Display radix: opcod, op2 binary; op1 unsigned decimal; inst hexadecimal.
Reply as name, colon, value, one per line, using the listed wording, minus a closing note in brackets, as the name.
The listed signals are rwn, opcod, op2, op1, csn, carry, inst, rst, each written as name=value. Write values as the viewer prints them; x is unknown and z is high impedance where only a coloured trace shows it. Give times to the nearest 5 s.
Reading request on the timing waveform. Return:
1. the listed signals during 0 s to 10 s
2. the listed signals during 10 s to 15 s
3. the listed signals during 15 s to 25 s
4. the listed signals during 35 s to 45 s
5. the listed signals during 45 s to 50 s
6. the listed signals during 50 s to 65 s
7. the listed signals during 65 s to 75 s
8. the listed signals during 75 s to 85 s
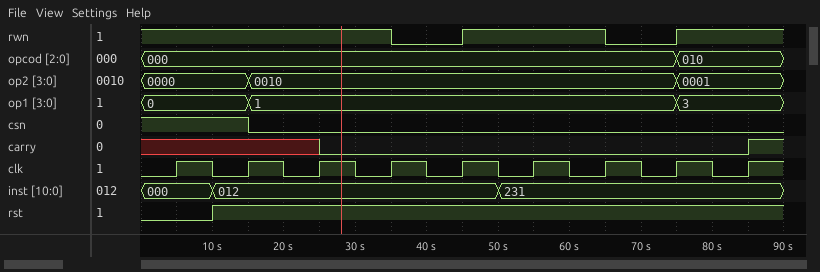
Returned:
the listed signals during 0 s to 10 s: rwn=1, opcod=000, op2=0000, op1=0, csn=1, carry=x, inst=000, rst=0
the listed signals during 10 s to 15 s: rwn=1, opcod=000, op2=0000, op1=0, csn=1, carry=x, inst=012, rst=1
the listed signals during 15 s to 25 s: rwn=1, opcod=000, op2=0010, op1=1, csn=0, carry=x, inst=012, rst=1
the listed signals during 35 s to 45 s: rwn=0, opcod=000, op2=0010, op1=1, csn=0, carry=0, inst=012, rst=1
the listed signals during 45 s to 50 s: rwn=1, opcod=000, op2=0010, op1=1, csn=0, carry=0, inst=012, rst=1
the listed signals during 50 s to 65 s: rwn=1, opcod=000, op2=0010, op1=1, csn=0, carry=0, inst=231, rst=1
the listed signals during 65 s to 75 s: rwn=0, opcod=000, op2=0010, op1=1, csn=0, carry=0, inst=231, rst=1
the listed signals during 75 s to 85 s: rwn=1, opcod=010, op2=0001, op1=3, csn=0, carry=0, inst=231, rst=1
